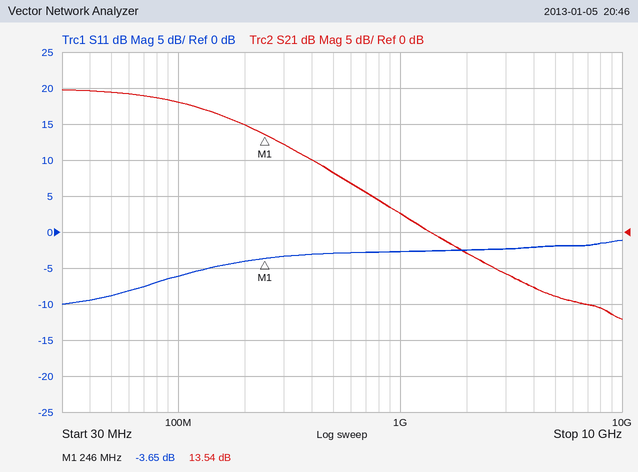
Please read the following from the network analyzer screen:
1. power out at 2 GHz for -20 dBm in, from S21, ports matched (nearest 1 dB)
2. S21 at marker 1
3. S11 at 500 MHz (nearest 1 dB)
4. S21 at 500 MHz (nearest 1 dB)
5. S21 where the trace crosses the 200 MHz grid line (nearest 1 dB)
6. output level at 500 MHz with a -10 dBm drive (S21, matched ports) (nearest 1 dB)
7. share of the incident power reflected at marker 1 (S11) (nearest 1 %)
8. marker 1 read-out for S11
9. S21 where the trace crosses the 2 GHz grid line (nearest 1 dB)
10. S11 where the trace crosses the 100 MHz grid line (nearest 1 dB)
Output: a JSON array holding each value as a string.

["-23 dBm", "13.54 dB", "-3 dB", "8 dB", "15 dB", "-2 dBm", "43 %", "-3.65 dB", "-3 dB", "-6 dB"]
